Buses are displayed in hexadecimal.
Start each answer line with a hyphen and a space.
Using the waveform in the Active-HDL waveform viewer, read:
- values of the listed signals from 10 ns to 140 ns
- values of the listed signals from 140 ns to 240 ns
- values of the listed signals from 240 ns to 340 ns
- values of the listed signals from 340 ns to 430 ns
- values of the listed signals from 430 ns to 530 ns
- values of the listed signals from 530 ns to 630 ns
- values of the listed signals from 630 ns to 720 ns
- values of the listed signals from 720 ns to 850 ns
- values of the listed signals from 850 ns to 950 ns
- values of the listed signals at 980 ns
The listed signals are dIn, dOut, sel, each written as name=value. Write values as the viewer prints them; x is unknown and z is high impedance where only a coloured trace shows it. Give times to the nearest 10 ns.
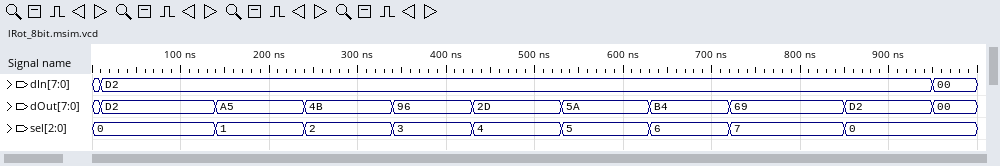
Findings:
- dIn=D2, dOut=D2, sel=0
- dIn=D2, dOut=A5, sel=1
- dIn=D2, dOut=4B, sel=2
- dIn=D2, dOut=96, sel=3
- dIn=D2, dOut=2D, sel=4
- dIn=D2, dOut=5A, sel=5
- dIn=D2, dOut=B4, sel=6
- dIn=D2, dOut=69, sel=7
- dIn=D2, dOut=D2, sel=0
- dIn=00, dOut=00, sel=0
